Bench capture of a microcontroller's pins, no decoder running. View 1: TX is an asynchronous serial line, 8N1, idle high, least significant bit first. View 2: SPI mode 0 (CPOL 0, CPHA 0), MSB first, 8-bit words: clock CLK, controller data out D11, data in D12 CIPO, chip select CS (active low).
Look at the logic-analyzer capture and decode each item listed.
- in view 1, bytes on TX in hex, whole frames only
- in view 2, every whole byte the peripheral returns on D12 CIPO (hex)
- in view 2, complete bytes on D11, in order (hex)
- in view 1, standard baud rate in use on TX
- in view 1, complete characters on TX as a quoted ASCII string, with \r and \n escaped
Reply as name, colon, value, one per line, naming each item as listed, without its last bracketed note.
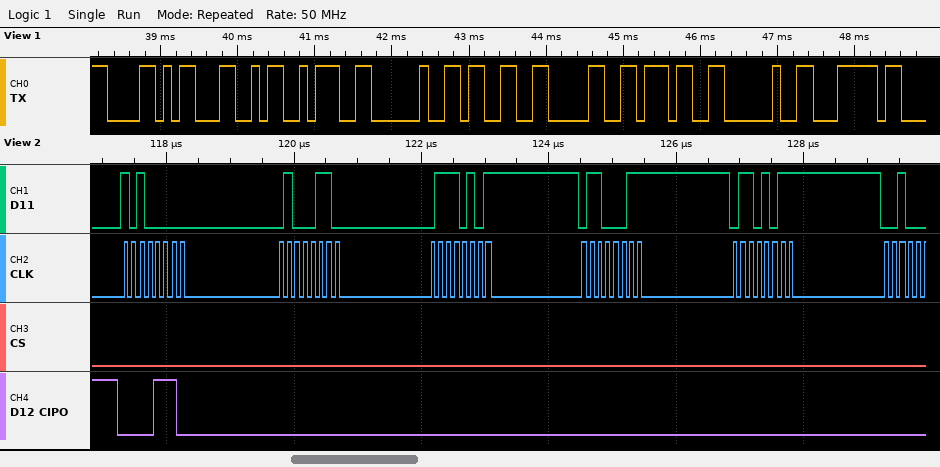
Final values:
in view 1, bytes on TX in hex, whole frames only: 0x58 0x4C 0x3A 0x20 0x33 0x30 0x37 0x20 0x7C
in view 2, every whole byte the peripheral returns on D12 CIPO: 0E 00 00 00 00
in view 2, complete bytes on D11, in order: A0 46 75 63 6B
in view 1, standard baud rate in use on TX: 9600 baud
in view 1, complete characters on TX as a quoted ASCII string, with \r and \n escaped: "XL: 307 |"
